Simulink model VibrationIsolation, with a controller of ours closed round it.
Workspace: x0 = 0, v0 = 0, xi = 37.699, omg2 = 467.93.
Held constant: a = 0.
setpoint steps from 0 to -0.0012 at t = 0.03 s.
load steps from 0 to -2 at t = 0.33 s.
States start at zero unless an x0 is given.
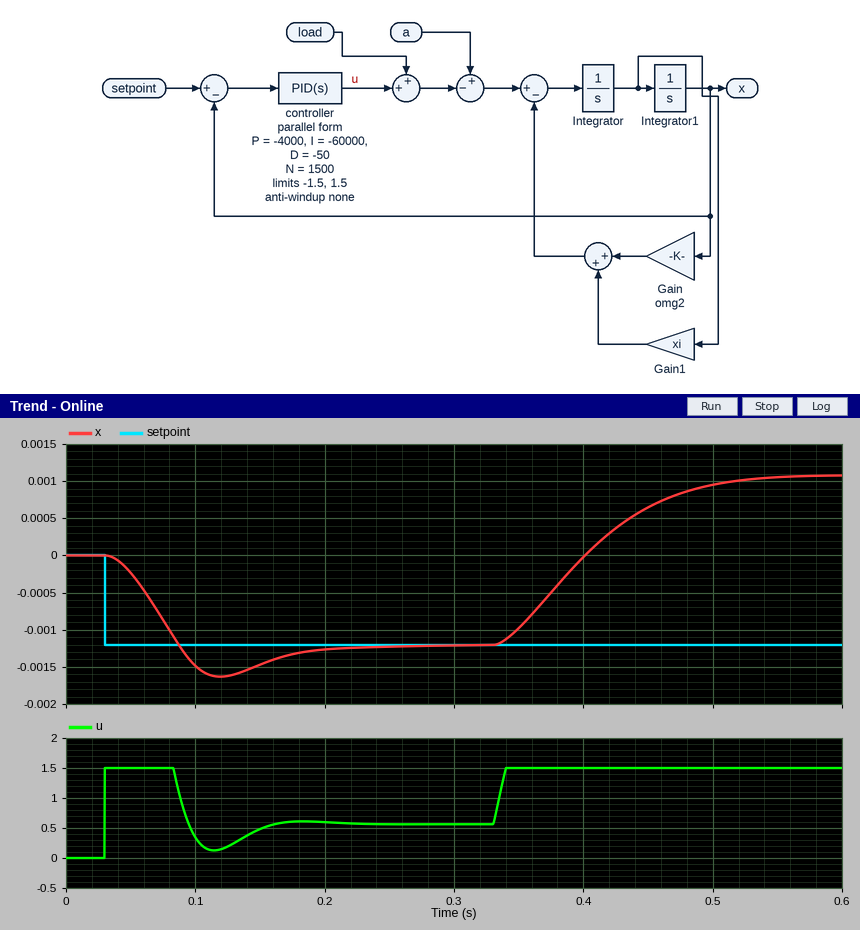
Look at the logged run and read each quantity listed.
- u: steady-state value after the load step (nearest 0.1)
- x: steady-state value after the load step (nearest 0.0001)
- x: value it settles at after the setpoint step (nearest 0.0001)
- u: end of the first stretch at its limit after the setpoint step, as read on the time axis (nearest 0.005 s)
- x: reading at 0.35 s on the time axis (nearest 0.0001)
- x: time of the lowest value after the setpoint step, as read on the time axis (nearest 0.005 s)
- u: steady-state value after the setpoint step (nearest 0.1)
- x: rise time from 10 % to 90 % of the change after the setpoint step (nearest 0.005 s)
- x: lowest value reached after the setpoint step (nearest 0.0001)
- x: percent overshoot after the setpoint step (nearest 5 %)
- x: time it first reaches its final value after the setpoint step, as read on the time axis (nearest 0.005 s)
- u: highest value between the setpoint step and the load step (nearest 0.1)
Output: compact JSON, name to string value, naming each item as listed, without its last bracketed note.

{"u: steady-state value after the load step": "1.5", "x: steady-state value after the load step": "0.0011", "x: value it settles at after the setpoint step": "-0.0012", "u: end of the first stretch at its limit after the setpoint step, as read on the time axis": "0.085 s", "x: reading at 0.35 s on the time axis": "-0.0010", "x: time of the lowest value after the setpoint step, as read on the time axis": "0.120 s", "u: steady-state value after the setpoint step": "0.6", "x: rise time from 10 % to 90 % of the change after the setpoint step": "0.040 s", "x: lowest value reached after the setpoint step": "-0.0016", "x: percent overshoot after the setpoint step": "35 %", "x: time it first reaches its final value after the setpoint step, as read on the time axis": "0.085 s", "u: highest value between the setpoint step and the load step": "1.5"}
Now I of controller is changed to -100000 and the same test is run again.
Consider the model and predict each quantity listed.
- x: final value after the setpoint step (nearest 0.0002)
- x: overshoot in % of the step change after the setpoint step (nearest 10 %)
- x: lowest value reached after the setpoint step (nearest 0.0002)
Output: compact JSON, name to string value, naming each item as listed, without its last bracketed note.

{"x: final value after the setpoint step": "-0.0012", "x: overshoot in % of the step change after the setpoint step": "60 %", "x: lowest value reached after the setpoint step": "-0.0018"}
